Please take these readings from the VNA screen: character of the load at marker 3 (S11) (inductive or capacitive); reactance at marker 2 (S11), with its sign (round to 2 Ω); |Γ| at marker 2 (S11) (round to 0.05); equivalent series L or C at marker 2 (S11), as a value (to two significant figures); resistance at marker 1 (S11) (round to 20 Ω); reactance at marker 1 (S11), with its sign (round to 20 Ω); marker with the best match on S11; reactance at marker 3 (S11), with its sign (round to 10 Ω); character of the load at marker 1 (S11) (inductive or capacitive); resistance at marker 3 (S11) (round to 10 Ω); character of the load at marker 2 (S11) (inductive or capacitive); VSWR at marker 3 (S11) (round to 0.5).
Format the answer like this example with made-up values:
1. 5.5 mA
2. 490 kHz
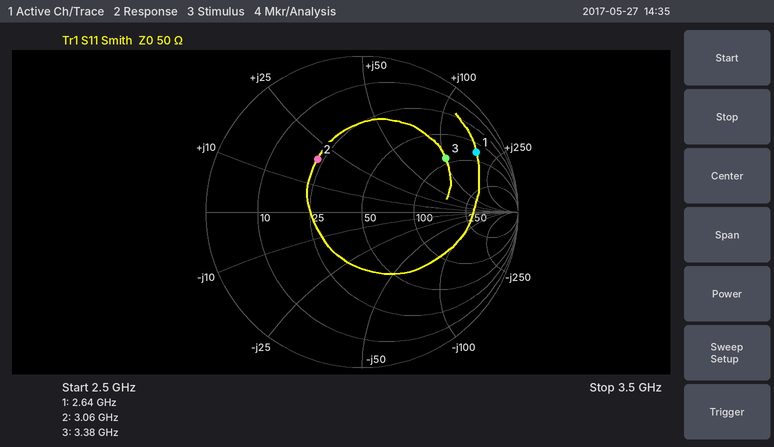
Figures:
1. inductive
2. +20 Ω
3. 0.45
4. 1.0 nH
5. 80 Ω
6. +180 Ω
7. marker 2
8. +100 Ω
9. inductive
10. 90 Ω
11. inductive
12. 4.5
